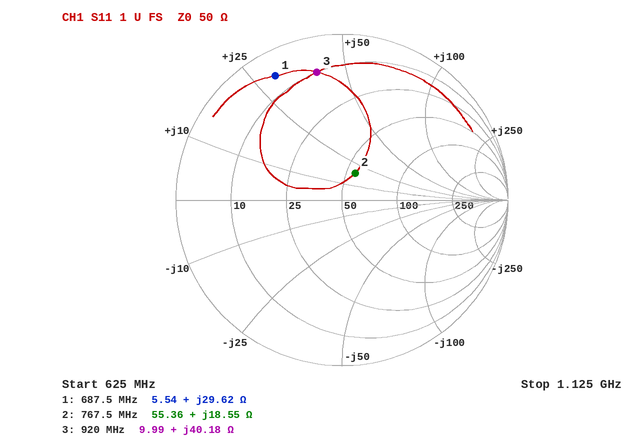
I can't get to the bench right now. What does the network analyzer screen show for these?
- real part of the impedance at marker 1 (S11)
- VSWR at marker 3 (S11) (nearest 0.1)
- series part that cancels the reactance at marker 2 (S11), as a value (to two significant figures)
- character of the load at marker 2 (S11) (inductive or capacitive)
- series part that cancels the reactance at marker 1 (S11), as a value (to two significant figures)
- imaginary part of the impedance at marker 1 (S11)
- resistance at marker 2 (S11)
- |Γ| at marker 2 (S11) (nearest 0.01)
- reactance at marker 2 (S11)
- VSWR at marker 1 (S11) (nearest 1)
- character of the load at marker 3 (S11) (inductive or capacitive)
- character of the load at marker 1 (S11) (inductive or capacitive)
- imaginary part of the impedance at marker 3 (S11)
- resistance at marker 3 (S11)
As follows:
5.54 Ω
8.3
11 pF
inductive
7.8 pF
+29.62 Ω
55.36 Ω
0.18
+18.55 Ω
12
inductive
inductive
+40.18 Ω
9.99 Ω
